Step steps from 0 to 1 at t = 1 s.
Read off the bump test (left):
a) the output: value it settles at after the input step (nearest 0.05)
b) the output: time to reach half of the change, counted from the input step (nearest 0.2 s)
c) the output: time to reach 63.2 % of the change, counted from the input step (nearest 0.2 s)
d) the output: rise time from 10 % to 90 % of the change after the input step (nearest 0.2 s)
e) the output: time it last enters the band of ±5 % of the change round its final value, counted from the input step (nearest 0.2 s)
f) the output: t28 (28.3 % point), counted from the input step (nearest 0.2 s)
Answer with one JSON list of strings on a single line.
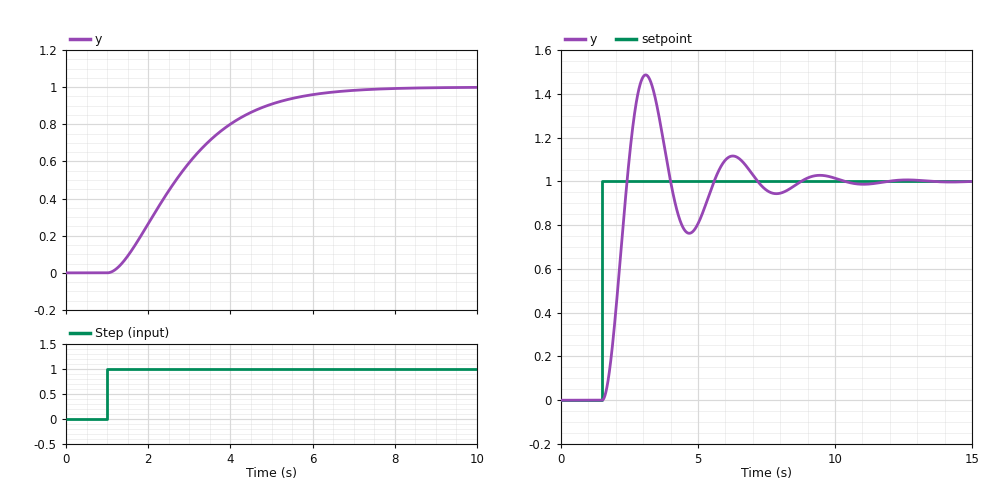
["1.00", "1.6 s", "2.2 s", "3.4 s", "4.8 s", "1.0 s"]
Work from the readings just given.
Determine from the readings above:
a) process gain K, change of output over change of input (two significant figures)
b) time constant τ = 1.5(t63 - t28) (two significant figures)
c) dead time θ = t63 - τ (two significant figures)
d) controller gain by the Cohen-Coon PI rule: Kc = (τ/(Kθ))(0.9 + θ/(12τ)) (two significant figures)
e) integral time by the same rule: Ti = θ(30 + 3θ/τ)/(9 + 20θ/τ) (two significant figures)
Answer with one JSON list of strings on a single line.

["1.0", "1.8 s", "0.40 s", "4.1", "0.91 s"]
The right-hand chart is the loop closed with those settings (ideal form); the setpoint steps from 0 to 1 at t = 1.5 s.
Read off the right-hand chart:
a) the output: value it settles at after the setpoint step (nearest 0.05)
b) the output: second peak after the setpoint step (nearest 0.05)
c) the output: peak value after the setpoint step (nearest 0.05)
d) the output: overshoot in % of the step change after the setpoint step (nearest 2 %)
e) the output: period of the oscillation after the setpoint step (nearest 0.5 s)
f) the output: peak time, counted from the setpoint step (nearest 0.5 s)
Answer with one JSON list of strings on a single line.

["1.00", "1.10", "1.50", "48 %", "3.0 s", "1.5 s"]
